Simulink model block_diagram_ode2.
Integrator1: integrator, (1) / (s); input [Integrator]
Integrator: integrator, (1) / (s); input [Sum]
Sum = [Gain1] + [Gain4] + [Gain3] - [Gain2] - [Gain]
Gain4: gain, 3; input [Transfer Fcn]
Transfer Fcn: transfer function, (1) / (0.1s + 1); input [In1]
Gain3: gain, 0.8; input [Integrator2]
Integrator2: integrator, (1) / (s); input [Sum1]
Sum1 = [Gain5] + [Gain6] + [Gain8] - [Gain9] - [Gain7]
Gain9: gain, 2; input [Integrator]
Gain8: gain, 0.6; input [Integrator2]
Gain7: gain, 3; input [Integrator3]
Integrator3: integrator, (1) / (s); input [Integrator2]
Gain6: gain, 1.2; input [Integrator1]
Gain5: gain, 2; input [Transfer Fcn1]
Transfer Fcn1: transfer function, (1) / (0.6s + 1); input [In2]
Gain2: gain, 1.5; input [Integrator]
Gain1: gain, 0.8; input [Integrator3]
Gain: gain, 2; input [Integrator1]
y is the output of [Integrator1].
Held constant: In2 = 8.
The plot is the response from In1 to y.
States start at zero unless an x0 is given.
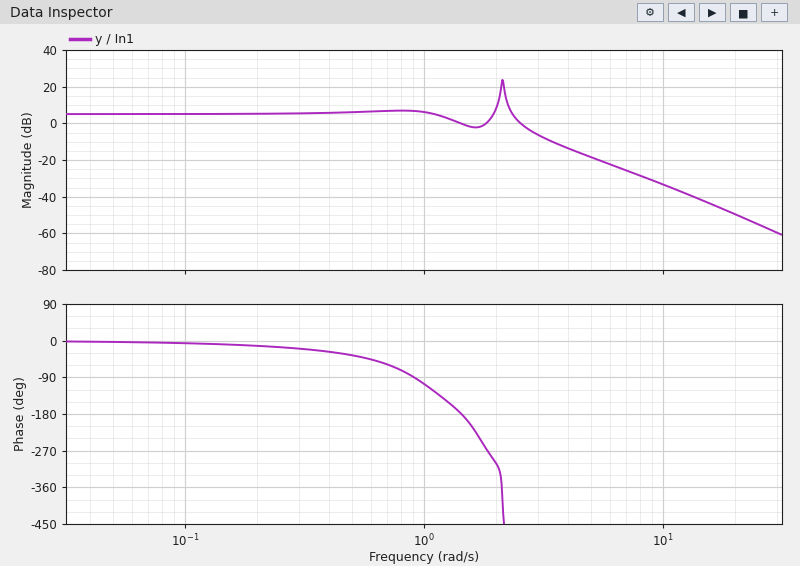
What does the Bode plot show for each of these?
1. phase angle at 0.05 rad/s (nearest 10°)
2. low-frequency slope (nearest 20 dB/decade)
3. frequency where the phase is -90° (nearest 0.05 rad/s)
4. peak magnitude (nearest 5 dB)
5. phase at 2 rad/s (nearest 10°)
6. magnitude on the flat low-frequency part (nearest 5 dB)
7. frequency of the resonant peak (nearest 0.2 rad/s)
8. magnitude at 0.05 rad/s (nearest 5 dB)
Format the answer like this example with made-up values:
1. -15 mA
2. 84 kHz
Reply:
1. 0°
2. 0 dB/decade
3. 0.90 rad/s
4. 25 dB
5. -300°
6. 5 dB
7. 2.2 rad/s
8. 5 dB
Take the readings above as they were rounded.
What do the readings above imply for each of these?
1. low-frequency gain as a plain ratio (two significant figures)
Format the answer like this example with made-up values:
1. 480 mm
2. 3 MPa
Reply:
1. 1.8
